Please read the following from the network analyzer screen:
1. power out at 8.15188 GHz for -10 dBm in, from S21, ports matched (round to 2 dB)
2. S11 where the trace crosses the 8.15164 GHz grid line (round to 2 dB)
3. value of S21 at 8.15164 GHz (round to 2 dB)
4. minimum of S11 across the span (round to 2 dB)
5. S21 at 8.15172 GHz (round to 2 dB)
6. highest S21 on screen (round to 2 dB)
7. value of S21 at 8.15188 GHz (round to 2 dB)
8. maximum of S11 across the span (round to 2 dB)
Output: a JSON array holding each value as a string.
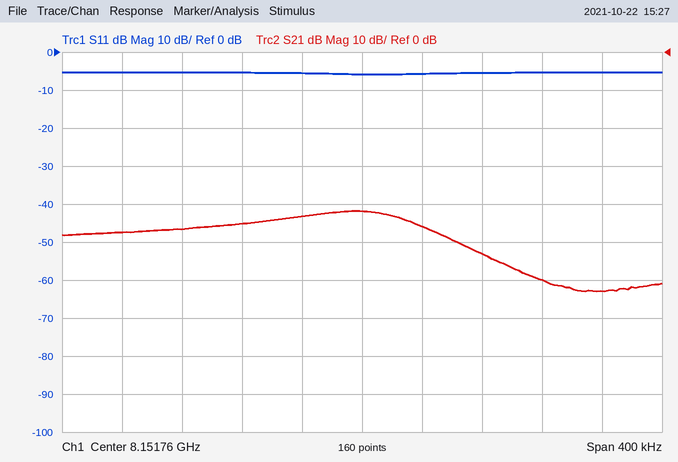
["-70 dBm", "-6 dB", "-46 dB", "-6 dB", "-44 dB", "-42 dB", "-60 dB", "-6 dB"]
